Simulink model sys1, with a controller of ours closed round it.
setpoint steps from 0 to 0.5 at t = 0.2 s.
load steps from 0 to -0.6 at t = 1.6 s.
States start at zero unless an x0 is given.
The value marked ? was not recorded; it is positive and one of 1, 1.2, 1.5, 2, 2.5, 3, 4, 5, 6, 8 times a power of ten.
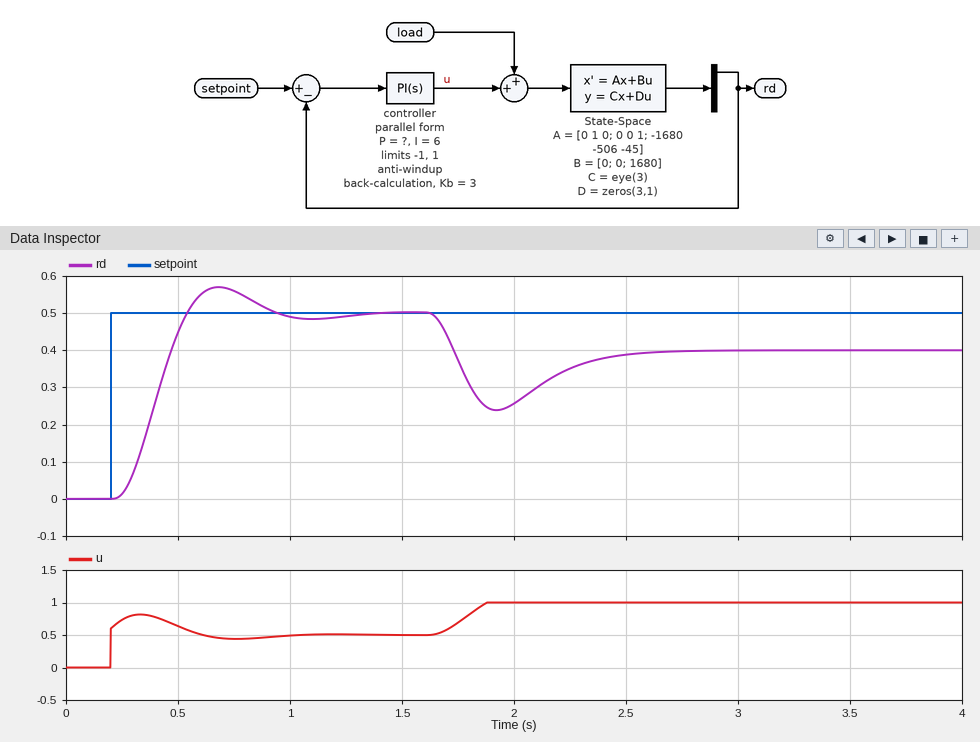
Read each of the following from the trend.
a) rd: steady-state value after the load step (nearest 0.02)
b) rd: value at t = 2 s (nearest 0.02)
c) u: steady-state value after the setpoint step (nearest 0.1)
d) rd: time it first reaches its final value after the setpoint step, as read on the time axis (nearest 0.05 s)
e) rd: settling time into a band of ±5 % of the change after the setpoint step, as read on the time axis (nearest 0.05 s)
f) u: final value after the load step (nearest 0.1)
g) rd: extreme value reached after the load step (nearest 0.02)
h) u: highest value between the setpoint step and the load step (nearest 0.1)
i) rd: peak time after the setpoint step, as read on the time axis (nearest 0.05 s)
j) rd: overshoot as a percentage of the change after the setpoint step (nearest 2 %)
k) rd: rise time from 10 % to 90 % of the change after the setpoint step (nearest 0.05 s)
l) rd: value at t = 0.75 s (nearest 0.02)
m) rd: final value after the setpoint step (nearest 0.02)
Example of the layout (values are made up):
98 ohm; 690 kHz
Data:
0.40; 0.26; 0.5; 0.55 s; 0.85 s; 1.0; 0.24; 0.8; 0.70 s; 14 %; 0.20 s; 0.56; 0.50
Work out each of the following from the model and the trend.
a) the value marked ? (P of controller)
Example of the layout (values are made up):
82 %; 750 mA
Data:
1.2
